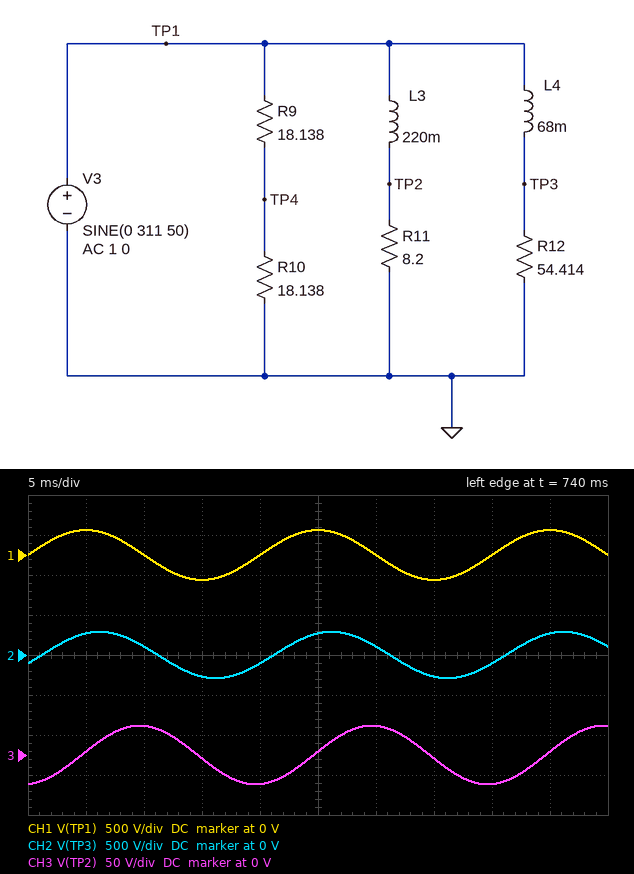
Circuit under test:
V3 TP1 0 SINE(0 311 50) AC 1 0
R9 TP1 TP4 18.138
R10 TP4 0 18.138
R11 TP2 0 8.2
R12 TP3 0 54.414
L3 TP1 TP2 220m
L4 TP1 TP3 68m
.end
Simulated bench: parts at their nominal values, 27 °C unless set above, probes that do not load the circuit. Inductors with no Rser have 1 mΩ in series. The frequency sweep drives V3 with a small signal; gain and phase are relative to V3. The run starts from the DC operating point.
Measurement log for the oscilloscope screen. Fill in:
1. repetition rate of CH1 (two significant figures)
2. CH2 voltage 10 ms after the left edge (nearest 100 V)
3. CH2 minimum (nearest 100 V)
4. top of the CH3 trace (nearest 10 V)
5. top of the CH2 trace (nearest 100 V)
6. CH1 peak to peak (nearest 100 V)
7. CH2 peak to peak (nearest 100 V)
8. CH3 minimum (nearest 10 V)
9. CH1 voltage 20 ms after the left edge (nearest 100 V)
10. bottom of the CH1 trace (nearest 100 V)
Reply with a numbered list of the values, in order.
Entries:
1. 50 Hz
2. 100 V
3. -300 V
4. 40 V
5. 300 V
6. 600 V
7. 600 V
8. -40 V
9. 0 V
10. -300 V
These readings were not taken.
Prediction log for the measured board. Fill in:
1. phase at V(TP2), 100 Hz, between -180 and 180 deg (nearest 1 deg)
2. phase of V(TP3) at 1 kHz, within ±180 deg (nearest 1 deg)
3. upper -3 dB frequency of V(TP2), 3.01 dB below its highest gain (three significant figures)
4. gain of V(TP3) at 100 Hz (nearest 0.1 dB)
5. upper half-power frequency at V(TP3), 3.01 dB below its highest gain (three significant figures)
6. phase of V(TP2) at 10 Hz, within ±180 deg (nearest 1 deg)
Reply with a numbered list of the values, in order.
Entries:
1. -87 deg
2. -83 deg
3. 5.93 Hz
4. -2.1 dB
5. 127 Hz
6. -59 deg
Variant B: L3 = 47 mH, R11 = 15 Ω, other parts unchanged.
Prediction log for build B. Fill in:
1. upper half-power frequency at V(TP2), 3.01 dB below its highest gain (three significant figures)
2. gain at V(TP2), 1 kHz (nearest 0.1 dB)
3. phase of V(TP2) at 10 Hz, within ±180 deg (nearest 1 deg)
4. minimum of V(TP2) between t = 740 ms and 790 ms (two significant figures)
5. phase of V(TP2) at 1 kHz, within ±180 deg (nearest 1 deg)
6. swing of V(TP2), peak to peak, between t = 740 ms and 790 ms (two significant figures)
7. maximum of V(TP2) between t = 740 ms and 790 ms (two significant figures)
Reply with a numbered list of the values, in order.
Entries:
1. 50.8 Hz
2. -25.9 dB
3. -11 deg
4. -220 V
5. -87 deg
6. 440 V
7. 220 V
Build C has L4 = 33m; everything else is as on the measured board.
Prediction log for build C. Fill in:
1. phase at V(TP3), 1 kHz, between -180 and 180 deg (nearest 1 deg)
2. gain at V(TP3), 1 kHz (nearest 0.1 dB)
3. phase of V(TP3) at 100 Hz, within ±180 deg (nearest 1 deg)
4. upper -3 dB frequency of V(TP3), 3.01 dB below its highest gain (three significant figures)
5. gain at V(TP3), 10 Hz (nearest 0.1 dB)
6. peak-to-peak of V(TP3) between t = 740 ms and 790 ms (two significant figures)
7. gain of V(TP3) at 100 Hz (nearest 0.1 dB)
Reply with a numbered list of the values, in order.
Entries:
1. -75 deg
2. -11.9 dB
3. -21 deg
4. 262 Hz
5. 0 dB
6. 610 V
7. -0.6 dB
